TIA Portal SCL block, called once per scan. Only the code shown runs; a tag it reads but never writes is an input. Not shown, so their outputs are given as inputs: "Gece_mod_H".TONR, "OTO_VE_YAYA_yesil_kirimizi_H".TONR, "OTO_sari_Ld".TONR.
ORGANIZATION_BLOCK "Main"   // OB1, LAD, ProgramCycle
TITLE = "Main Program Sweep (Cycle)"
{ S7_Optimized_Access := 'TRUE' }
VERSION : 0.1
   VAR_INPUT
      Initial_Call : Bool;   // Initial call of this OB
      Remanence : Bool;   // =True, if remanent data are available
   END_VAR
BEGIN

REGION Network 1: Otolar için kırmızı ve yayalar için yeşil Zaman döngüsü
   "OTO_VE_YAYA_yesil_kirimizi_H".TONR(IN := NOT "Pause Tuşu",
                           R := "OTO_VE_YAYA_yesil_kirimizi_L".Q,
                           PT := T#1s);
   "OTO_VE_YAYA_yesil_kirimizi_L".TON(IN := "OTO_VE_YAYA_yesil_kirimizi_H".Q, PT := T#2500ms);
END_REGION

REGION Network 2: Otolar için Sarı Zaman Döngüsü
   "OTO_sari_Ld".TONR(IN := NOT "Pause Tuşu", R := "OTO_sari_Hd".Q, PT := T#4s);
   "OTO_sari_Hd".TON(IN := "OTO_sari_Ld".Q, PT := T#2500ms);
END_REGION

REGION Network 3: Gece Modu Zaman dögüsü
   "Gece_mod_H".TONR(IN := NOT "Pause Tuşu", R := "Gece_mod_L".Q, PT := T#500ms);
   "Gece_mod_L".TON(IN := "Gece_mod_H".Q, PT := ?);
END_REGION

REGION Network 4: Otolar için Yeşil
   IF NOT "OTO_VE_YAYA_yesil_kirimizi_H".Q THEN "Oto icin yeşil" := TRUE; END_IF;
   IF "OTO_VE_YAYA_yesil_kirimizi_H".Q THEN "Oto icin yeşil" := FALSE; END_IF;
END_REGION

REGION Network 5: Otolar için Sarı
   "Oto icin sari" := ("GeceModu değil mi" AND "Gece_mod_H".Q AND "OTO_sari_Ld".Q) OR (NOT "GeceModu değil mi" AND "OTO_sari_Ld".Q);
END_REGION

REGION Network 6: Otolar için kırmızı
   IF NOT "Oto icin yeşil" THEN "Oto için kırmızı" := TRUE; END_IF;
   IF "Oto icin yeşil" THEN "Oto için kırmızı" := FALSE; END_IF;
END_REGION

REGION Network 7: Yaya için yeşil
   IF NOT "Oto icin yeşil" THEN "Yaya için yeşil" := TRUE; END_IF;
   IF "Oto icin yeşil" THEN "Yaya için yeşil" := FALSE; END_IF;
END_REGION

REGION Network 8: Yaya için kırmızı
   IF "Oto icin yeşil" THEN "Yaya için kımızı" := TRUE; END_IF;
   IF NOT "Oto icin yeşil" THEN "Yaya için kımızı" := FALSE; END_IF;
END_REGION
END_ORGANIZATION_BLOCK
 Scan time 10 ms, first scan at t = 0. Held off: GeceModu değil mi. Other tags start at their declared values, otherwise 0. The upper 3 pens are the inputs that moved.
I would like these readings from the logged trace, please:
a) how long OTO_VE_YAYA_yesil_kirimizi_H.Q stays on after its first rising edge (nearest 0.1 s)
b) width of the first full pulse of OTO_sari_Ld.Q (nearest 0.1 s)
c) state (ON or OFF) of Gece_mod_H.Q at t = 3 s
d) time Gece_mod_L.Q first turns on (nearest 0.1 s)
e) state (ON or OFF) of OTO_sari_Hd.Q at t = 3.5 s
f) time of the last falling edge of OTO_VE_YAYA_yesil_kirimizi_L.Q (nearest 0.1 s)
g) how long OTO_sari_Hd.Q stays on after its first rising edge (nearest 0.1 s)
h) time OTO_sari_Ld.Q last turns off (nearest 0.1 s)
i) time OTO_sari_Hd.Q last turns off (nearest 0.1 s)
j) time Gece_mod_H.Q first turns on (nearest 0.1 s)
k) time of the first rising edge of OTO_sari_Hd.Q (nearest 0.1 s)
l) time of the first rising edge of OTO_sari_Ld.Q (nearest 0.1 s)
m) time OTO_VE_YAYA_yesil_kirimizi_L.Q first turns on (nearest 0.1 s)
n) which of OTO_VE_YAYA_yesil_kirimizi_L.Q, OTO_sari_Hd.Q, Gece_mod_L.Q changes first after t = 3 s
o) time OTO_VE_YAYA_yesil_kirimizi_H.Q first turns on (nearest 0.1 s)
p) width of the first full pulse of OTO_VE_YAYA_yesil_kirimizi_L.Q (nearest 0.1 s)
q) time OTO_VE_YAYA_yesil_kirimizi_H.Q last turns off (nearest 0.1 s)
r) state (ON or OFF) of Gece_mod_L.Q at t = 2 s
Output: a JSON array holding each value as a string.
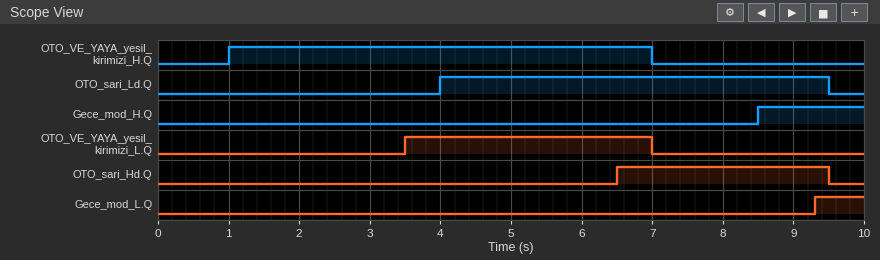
["6.0 s", "5.5 s", "OFF", "9.3 s", "OFF", "7.0 s", "3.0 s", "9.5 s", "9.5 s", "8.5 s", "6.5 s", "4.0 s", "3.5 s", "OTO_VE_YAYA_yesil_kirimizi_L.Q", "1.0 s", "3.5 s", "7.0 s", "OFF"]
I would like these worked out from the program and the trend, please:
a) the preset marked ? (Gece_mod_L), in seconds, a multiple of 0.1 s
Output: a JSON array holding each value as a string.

["0.8 s"]
